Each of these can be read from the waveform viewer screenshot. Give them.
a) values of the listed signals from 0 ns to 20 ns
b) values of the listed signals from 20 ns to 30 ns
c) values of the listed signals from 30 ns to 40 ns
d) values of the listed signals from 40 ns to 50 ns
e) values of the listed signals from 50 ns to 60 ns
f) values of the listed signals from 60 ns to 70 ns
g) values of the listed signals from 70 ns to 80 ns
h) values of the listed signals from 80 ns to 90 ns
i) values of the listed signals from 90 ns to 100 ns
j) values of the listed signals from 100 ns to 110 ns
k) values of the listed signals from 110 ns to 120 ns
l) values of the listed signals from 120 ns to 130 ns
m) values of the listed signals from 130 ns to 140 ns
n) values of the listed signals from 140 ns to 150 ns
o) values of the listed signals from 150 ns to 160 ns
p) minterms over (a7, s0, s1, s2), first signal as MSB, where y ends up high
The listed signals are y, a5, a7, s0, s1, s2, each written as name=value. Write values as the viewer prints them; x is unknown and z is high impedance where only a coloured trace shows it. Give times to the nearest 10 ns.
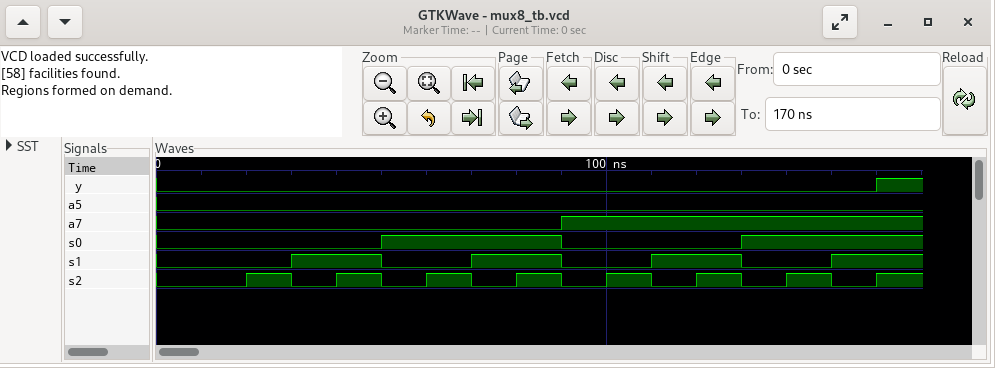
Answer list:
y=0, a5=0, a7=0, s0=0, s1=0, s2=0
y=0, a5=0, a7=0, s0=0, s1=0, s2=1
y=0, a5=0, a7=0, s0=0, s1=1, s2=0
y=0, a5=0, a7=0, s0=0, s1=1, s2=1
y=0, a5=0, a7=0, s0=1, s1=0, s2=0
y=0, a5=0, a7=0, s0=1, s1=0, s2=1
y=0, a5=0, a7=0, s0=1, s1=1, s2=0
y=0, a5=0, a7=0, s0=1, s1=1, s2=1
y=0, a5=0, a7=1, s0=0, s1=0, s2=0
y=0, a5=0, a7=1, s0=0, s1=0, s2=1
y=0, a5=0, a7=1, s0=0, s1=1, s2=0
y=0, a5=0, a7=1, s0=0, s1=1, s2=1
y=0, a5=0, a7=1, s0=1, s1=0, s2=0
y=0, a5=0, a7=1, s0=1, s1=0, s2=1
y=0, a5=0, a7=1, s0=1, s1=1, s2=0
15
